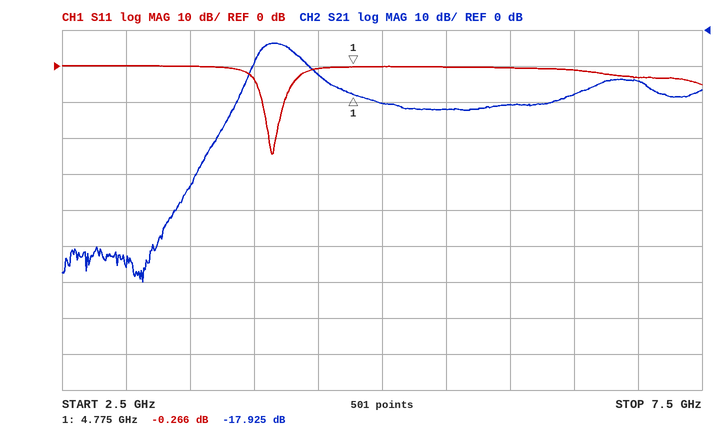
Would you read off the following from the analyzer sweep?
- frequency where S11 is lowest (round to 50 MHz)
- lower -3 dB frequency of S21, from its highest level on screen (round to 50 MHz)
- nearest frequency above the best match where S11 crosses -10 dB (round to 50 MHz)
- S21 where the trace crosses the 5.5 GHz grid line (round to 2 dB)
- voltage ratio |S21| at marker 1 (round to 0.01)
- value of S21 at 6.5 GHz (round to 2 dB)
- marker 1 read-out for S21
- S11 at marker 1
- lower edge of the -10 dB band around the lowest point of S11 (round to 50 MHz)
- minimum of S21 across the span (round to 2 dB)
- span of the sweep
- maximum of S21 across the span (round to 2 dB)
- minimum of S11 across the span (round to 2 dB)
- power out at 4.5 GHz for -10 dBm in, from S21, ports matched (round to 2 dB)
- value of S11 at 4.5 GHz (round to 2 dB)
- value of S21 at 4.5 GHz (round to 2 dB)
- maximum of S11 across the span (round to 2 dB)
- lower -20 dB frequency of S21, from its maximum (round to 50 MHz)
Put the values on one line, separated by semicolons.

4.15 GHz; 4.05 GHz; 4.25 GHz; -22 dB; 0.13; -18 dB; -17.925 dB; -0.266 dB; 4.05 GHz; -70 dB; 5 GHz; -4 dB; -24 dB; -22 dBm; 0 dB; -12 dB; 0 dB; 3.80 GHz
